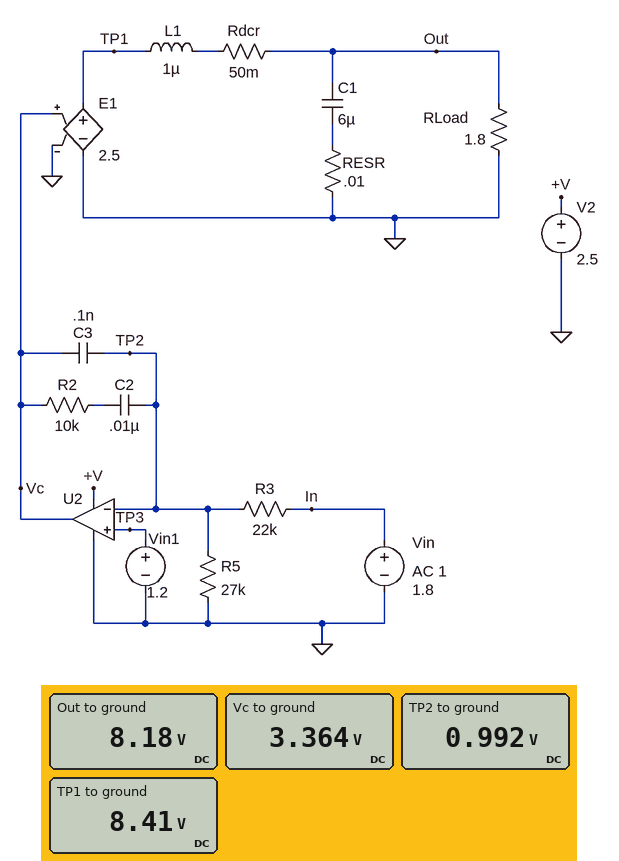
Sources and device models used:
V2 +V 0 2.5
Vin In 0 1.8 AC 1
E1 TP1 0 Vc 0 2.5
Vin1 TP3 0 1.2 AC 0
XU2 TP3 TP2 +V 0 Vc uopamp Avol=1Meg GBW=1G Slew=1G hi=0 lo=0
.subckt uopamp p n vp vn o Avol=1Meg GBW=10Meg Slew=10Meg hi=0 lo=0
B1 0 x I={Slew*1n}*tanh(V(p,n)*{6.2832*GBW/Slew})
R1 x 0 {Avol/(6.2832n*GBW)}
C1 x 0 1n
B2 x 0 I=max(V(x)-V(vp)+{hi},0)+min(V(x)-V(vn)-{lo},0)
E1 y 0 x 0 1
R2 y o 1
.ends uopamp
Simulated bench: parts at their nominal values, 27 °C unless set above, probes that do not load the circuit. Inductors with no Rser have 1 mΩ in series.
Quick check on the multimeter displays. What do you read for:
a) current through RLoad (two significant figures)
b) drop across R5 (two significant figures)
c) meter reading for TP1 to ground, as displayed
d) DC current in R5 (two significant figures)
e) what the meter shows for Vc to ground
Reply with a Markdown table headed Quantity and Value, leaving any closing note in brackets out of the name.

| Quantity | Value |
|---|---|
| current through RLoad | 4.5 A |
| drop across R5 | 990 mV |
| meter reading for TP1 to ground, as displayed | 8.41 V |
| DC current in R5 | 37 µA |
| what the meter shows for Vc to ground | 3.364 V |
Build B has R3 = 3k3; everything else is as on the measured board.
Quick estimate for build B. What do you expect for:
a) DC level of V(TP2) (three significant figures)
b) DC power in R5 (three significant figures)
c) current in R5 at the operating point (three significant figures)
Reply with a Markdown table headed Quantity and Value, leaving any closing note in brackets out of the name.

| Quantity | Value |
|---|---|
| DC level of V(TP2) | 1.60 V |
| DC power in R5 | 95.3 µW |
| current in R5 at the operating point | 59.4 µA |
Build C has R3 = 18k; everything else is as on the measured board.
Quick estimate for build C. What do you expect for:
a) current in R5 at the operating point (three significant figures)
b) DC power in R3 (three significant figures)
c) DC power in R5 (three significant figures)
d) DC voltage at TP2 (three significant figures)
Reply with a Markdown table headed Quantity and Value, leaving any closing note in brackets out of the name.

| Quantity | Value |
|---|---|
| current in R5 at the operating point | 40.0 µA |
| DC power in R3 | 28.8 µW |
| DC power in R5 | 43.2 µW |
| DC voltage at TP2 | 1.08 V |
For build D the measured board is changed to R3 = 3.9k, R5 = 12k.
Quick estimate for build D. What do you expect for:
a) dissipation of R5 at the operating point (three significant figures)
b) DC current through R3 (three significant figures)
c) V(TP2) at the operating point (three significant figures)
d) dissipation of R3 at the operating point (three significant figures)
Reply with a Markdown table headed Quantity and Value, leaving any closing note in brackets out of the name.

| Quantity | Value |
|---|---|
| dissipation of R5 at the operating point | 154 µW |
| DC current through R3 | 113 µA |
| V(TP2) at the operating point | 1.36 V |
| dissipation of R3 at the operating point | 50.0 µW |
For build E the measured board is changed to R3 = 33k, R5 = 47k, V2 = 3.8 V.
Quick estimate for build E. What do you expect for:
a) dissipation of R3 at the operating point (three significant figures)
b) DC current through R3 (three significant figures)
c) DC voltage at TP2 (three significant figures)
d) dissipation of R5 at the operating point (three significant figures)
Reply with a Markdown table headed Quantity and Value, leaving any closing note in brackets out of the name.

| Quantity | Value |
|---|---|
| dissipation of R3 at the operating point | 16.7 µW |
| DC current through R3 | 22.5 µA |
| DC voltage at TP2 | 1.06 V |
| dissipation of R5 at the operating point | 23.8 µW |
